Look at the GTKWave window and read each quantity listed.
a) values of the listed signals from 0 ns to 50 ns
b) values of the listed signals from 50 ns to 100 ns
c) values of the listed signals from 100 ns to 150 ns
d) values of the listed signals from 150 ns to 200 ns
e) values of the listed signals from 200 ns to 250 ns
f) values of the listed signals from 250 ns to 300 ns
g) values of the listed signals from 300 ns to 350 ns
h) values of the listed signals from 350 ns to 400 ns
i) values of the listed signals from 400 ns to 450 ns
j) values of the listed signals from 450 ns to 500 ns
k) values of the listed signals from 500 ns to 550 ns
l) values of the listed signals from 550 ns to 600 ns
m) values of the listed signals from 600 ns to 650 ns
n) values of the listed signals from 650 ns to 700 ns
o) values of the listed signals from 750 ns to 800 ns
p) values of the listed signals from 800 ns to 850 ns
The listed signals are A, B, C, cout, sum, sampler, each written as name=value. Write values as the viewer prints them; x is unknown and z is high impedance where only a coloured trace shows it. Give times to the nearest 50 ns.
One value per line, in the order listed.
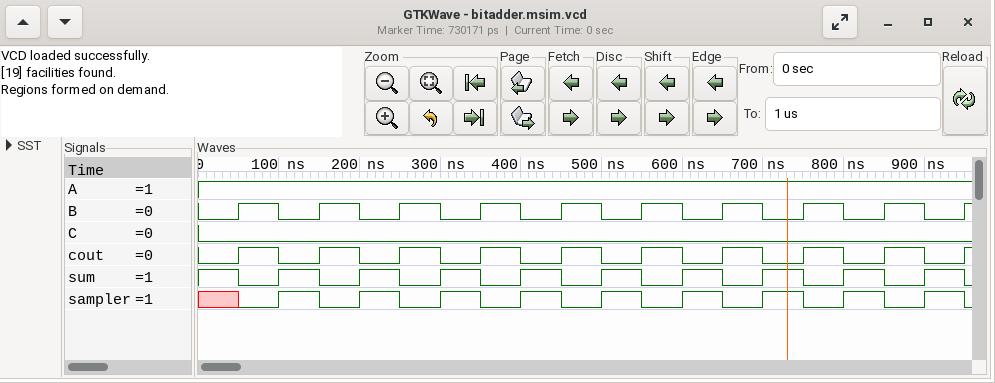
A=1, B=0, C=0, cout=0, sum=1, sampler=x
A=1, B=1, C=0, cout=1, sum=0, sampler=0
A=1, B=0, C=0, cout=0, sum=1, sampler=1
A=1, B=1, C=0, cout=1, sum=0, sampler=0
A=1, B=0, C=0, cout=0, sum=1, sampler=1
A=1, B=1, C=0, cout=1, sum=0, sampler=0
A=1, B=0, C=0, cout=0, sum=1, sampler=1
A=1, B=1, C=0, cout=1, sum=0, sampler=0
A=1, B=0, C=0, cout=0, sum=1, sampler=1
A=1, B=1, C=0, cout=1, sum=0, sampler=0
A=1, B=0, C=0, cout=0, sum=1, sampler=1
A=1, B=1, C=0, cout=1, sum=0, sampler=0
A=1, B=0, C=0, cout=0, sum=1, sampler=1
A=1, B=1, C=0, cout=1, sum=0, sampler=0
A=1, B=1, C=0, cout=1, sum=0, sampler=0
A=1, B=0, C=0, cout=0, sum=1, sampler=1
